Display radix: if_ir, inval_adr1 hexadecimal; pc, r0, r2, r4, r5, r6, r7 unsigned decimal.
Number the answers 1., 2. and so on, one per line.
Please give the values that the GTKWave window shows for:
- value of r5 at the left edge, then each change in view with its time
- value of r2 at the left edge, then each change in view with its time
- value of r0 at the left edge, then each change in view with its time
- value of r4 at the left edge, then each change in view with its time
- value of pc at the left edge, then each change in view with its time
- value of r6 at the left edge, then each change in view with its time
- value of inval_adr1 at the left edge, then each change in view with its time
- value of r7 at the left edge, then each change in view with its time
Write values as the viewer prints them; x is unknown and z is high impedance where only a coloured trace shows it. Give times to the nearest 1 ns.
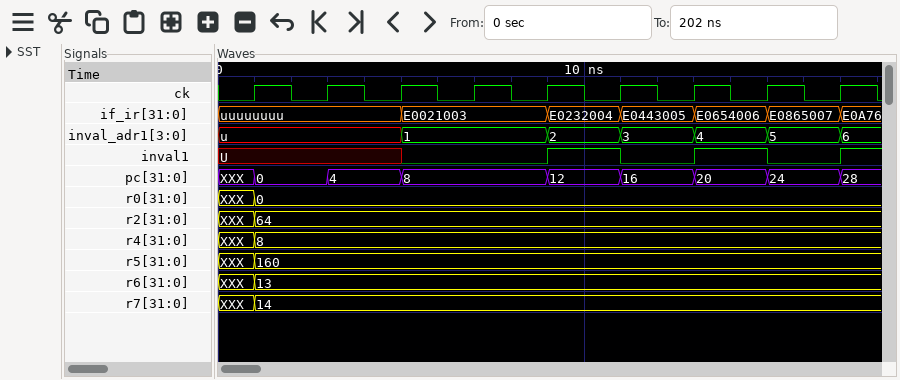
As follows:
1. XXX, 160 at 1 ns
2. XXX, 64 at 1 ns
3. XXX, 0 at 1 ns
4. XXX, 8 at 1 ns
5. XXX, 0 at 1 ns, 4 at 3 ns, 8 at 5 ns, 12 at 9 ns, 16 at 11 ns, 20 at 13 ns, 24 at 15 ns, 28 at 17 ns
6. XXX, 13 at 1 ns
7. u, 1 at 5 ns, 2 at 9 ns, 3 at 11 ns, 4 at 13 ns, 5 at 15 ns, 6 at 17 ns
8. XXX, 14 at 1 ns
